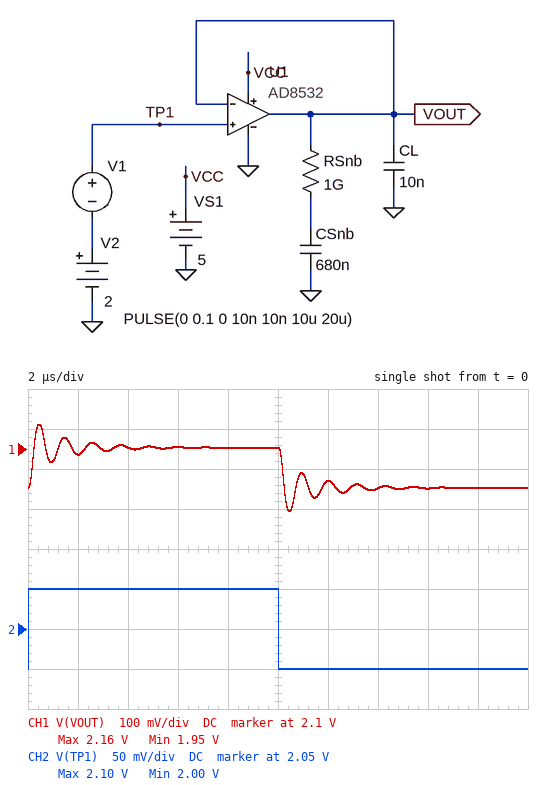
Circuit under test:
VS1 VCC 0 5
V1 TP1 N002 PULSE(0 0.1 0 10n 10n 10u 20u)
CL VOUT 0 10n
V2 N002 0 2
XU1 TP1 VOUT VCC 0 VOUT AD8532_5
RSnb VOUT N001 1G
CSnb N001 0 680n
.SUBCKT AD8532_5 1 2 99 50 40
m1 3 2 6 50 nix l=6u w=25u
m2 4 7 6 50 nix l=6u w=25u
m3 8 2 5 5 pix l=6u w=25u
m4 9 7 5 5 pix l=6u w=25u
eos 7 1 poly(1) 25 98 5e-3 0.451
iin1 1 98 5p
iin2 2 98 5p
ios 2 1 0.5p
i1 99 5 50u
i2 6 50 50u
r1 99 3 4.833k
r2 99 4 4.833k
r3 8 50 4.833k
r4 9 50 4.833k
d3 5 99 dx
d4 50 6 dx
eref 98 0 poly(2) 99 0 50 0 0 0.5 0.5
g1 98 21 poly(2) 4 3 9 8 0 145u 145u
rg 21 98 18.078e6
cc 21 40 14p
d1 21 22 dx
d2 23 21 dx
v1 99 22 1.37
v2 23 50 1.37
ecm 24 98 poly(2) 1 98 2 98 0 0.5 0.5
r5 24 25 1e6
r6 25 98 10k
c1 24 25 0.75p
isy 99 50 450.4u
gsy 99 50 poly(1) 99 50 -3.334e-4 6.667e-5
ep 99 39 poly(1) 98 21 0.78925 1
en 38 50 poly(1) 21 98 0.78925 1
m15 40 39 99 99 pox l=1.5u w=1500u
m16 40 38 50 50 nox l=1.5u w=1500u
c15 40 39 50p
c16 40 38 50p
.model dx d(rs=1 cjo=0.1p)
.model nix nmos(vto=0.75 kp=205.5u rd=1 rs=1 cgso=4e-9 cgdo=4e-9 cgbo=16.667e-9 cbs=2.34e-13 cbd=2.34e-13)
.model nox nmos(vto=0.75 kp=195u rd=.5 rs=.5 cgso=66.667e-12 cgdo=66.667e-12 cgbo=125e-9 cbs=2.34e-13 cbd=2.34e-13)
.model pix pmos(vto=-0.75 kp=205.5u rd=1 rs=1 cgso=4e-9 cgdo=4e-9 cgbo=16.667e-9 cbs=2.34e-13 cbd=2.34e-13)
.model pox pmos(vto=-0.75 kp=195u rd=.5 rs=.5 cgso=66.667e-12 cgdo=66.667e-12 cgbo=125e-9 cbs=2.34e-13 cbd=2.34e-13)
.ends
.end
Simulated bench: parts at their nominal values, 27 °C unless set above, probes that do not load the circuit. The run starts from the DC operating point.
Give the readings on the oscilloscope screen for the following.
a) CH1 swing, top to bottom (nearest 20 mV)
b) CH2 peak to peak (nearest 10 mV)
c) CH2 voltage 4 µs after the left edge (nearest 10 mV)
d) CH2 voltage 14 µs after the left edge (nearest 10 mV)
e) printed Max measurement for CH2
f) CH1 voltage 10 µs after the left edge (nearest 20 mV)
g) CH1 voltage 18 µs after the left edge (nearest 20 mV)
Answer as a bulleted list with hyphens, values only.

- 220 mV
- 100 mV
- 2.10 V
- 2.00 V
- 2.10 V
- 2.10 V
- 2.00 V
